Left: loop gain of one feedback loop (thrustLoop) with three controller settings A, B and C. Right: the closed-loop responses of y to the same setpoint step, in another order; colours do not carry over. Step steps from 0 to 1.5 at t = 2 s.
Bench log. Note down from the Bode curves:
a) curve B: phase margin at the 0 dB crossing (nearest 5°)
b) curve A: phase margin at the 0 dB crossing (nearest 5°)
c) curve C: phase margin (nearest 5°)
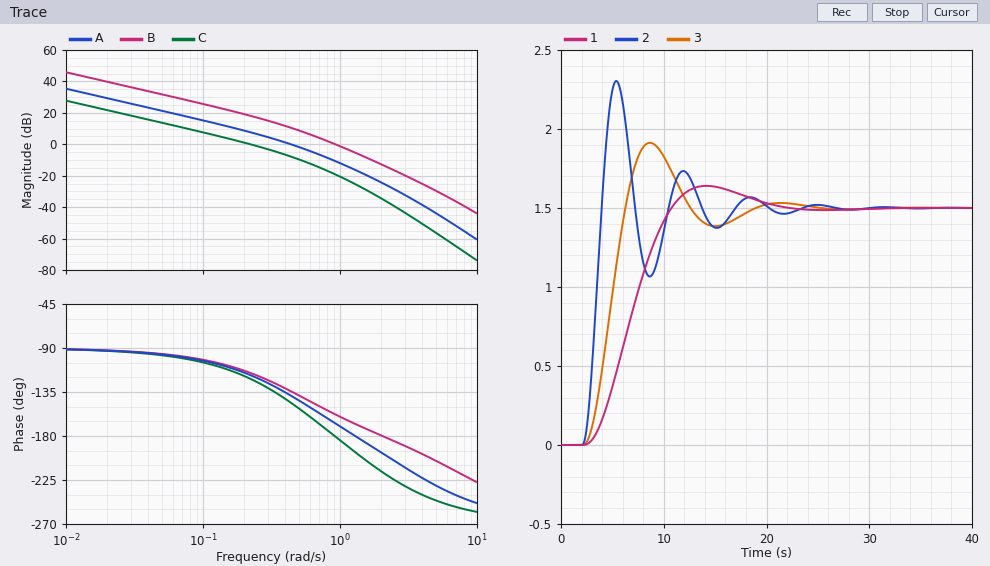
20°
40°
60°
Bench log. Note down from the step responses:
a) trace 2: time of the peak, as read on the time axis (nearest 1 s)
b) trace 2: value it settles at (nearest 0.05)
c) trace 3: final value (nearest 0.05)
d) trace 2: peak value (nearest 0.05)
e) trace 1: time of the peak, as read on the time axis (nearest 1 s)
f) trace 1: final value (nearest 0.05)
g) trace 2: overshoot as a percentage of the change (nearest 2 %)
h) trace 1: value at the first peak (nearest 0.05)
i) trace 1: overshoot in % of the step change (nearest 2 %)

5 s
1.50
1.50
2.30
14 s
1.50
54 %
1.65
10 %
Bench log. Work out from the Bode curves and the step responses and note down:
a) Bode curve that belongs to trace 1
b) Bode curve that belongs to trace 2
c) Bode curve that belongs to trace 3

C
B
A
